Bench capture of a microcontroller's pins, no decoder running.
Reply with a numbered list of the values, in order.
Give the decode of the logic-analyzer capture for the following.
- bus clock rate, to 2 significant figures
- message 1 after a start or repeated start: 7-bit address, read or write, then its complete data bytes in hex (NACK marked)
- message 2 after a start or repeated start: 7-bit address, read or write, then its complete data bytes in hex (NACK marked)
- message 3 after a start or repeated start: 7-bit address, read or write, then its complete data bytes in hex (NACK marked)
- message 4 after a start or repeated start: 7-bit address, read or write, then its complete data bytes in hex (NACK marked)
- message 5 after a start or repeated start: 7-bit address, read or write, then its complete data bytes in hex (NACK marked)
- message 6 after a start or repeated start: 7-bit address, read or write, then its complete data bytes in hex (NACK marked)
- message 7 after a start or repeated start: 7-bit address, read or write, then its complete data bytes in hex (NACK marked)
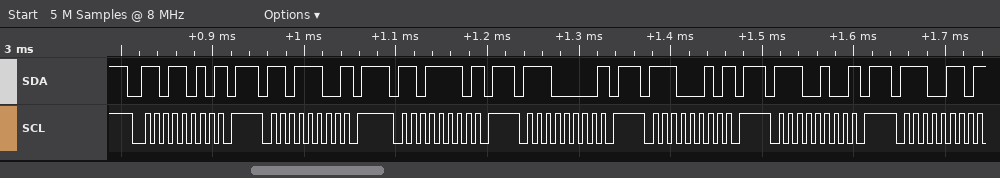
1. 100 kHz
2. 0x6D write NACK
3. 0x6E write NACK
4. 0x6F write NACK
5. 0x70 write NACK
6. 0x71 write NACK
7. 0x72 write NACK
8. 0x73 write NACK
